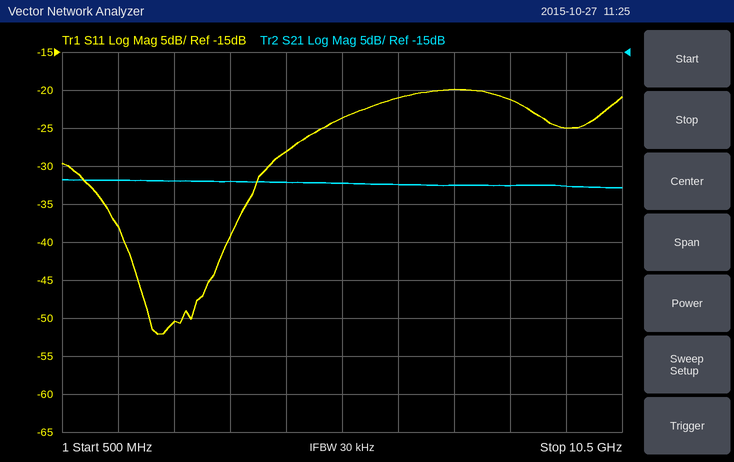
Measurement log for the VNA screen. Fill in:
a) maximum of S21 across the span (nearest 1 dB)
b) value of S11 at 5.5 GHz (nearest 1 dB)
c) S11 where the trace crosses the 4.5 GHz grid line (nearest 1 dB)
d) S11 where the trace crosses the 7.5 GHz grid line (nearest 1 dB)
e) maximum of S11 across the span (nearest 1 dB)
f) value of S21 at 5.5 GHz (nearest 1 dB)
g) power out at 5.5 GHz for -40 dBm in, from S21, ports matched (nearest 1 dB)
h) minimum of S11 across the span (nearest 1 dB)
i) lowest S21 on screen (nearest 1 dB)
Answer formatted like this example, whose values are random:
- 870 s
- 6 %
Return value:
- -32 dB
- -24 dB
- -28 dB
- -20 dB
- -20 dB
- -32 dB
- -72 dBm
- -52 dB
- -33 dB
